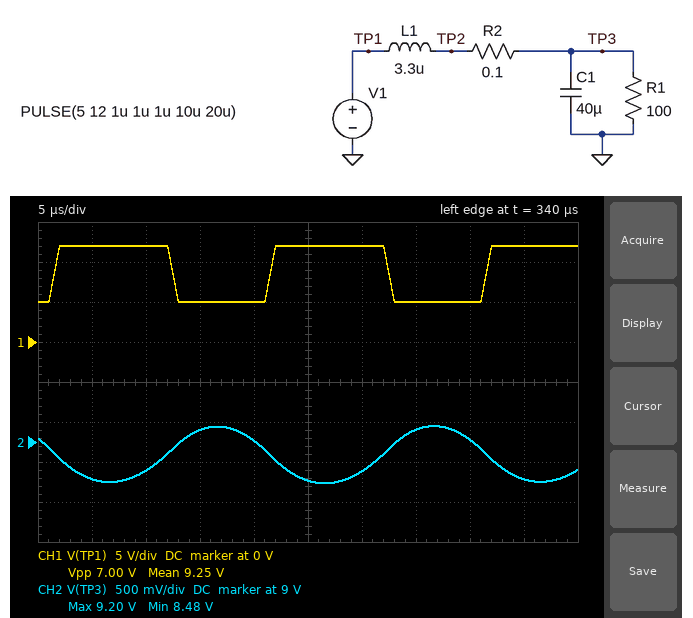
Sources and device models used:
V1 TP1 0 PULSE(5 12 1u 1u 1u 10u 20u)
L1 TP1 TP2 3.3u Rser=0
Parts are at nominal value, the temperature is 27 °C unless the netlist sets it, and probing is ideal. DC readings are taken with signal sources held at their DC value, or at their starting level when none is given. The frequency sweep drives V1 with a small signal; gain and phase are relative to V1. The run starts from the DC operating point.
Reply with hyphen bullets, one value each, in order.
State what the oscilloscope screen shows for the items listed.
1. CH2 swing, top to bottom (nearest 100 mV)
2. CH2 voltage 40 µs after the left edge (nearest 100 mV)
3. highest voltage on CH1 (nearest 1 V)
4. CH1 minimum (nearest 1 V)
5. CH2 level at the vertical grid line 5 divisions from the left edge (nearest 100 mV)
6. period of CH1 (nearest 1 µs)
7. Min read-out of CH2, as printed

- 700 mV
- 9.0 V
- 12 V
- 5 V
- 8.5 V
- 20 µs
- 8.48 V
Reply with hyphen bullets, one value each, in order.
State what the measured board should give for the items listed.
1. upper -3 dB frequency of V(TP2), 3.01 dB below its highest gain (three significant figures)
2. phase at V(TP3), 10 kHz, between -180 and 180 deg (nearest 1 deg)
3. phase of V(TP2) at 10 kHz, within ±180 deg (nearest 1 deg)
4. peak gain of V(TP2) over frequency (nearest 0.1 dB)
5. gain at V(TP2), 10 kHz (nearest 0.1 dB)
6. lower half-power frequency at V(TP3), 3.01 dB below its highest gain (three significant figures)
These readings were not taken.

- 15.8 kHz
- -28 deg
- -14 deg
- 9.7 dB
- 5.6 dB
- 10.7 kHz
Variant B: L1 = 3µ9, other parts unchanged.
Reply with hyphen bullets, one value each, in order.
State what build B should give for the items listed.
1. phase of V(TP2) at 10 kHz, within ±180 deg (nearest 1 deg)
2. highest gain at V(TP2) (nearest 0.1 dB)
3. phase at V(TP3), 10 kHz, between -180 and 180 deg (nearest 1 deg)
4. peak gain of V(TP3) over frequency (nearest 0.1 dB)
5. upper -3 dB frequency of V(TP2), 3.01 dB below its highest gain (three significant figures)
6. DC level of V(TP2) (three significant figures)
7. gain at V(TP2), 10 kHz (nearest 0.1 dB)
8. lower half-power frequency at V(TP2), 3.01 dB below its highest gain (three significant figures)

- -19 deg
- 10.3 dB
- -33 deg
- 9.9 dB
- 14.4 kHz
- 5.00 V
- 7.0 dB
- 10.2 kHz
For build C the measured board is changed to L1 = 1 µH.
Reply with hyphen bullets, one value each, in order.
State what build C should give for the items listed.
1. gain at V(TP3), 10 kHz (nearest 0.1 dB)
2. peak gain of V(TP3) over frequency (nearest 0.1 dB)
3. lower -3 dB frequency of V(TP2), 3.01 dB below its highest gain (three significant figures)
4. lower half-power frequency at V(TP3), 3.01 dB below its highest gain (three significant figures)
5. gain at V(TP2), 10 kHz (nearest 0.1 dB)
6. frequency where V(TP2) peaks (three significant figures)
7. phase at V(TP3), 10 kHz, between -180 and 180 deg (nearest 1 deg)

- 1.1 dB
- 4.4 dB
- 13.8 kHz
- 11.2 kHz
- 1.4 dB
- 23.3 kHz
- -17 deg
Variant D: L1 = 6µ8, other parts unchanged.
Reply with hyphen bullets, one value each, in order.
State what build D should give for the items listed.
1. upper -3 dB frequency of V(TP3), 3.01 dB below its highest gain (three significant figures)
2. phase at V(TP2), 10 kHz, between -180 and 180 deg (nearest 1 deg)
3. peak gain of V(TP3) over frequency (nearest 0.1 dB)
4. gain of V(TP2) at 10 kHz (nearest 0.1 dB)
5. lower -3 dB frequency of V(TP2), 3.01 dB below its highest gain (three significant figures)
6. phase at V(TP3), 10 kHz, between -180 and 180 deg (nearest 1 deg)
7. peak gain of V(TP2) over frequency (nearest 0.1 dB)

- 10.6 kHz
- -92 deg
- 12.2 dB
- 11.8 dB
- 8.24 kHz
- -106 deg
- 12.5 dB
